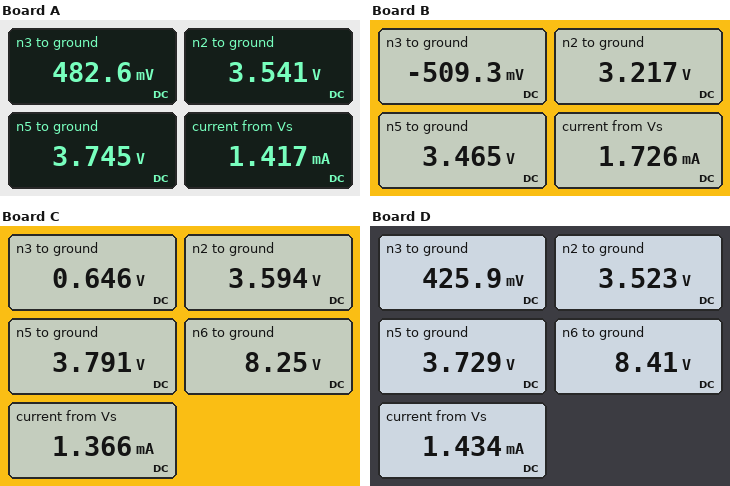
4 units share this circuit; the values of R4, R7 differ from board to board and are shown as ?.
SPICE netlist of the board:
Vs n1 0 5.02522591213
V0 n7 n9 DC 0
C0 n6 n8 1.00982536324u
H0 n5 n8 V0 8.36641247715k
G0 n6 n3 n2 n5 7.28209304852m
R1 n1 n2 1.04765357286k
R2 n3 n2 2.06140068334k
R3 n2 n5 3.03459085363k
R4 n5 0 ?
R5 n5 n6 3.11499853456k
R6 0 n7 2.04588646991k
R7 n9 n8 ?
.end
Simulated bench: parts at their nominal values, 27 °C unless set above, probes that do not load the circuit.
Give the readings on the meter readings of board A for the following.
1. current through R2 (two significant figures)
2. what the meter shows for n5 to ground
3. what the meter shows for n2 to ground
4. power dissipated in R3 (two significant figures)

1.5 mA
3.745 V
3.541 V
14 µW
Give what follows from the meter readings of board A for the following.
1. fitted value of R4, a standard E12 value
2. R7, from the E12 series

1.8 kΩ
680 Ω
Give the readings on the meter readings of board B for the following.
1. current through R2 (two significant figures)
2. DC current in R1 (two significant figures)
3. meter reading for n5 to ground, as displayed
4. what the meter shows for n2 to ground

1.8 mA
1.7 mA
3.465 V
3.217 V
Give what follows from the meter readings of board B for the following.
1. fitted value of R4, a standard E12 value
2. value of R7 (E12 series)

1.5 kΩ
390 Ω
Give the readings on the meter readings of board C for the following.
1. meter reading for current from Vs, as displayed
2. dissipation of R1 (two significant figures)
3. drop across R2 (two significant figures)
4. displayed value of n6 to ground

1.366 mA
2.0 mW
2.9 V
8.25 V
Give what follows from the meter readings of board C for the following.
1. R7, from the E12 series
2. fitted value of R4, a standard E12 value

1.2 kΩ
1.8 kΩ
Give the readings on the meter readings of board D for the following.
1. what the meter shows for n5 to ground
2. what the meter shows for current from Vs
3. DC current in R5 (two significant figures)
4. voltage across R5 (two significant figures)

3.729 V
1.434 mA
1.5 mA
4.7 V
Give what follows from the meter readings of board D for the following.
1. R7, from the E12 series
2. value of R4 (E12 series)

470 Ω
1.8 kΩ
